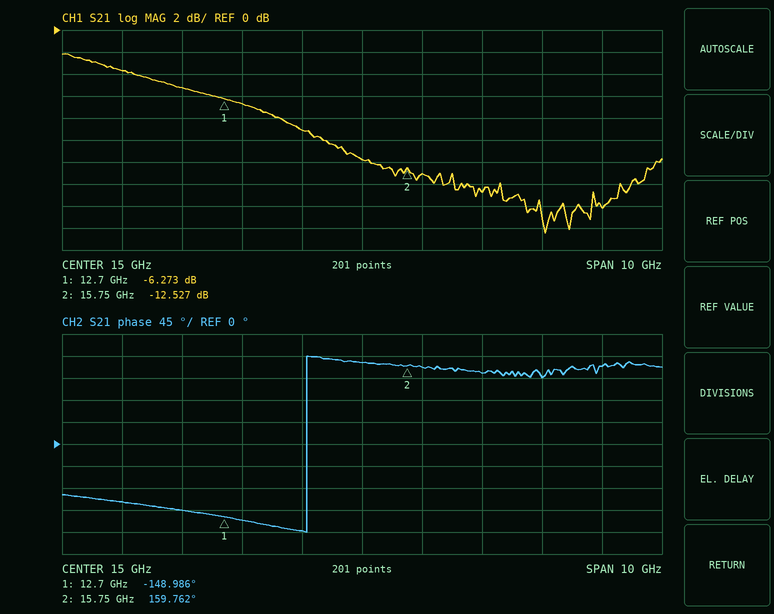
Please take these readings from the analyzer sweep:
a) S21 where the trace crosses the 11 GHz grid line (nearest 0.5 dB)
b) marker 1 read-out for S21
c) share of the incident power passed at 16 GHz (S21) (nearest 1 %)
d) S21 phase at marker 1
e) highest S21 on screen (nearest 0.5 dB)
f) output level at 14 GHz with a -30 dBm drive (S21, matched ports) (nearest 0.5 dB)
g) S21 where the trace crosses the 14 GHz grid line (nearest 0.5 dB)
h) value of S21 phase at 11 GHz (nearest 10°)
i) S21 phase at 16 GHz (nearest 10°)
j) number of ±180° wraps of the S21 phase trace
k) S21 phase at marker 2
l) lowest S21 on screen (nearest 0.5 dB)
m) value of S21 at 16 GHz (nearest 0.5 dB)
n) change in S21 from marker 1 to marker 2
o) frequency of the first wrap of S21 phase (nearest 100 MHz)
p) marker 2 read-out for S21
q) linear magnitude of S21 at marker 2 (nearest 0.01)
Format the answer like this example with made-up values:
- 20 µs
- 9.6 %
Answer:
- -3.5 dB
- -6.273 dB
- 5 %
- -148.986°
- -2.0 dB
- -39.0 dBm
- -9.0 dB
- -120°
- 160°
- 1
- 159.762°
- -18.5 dB
- -13.0 dB
- -6.254 dB
- 14.1 GHz
- -12.527 dB
- 0.24
